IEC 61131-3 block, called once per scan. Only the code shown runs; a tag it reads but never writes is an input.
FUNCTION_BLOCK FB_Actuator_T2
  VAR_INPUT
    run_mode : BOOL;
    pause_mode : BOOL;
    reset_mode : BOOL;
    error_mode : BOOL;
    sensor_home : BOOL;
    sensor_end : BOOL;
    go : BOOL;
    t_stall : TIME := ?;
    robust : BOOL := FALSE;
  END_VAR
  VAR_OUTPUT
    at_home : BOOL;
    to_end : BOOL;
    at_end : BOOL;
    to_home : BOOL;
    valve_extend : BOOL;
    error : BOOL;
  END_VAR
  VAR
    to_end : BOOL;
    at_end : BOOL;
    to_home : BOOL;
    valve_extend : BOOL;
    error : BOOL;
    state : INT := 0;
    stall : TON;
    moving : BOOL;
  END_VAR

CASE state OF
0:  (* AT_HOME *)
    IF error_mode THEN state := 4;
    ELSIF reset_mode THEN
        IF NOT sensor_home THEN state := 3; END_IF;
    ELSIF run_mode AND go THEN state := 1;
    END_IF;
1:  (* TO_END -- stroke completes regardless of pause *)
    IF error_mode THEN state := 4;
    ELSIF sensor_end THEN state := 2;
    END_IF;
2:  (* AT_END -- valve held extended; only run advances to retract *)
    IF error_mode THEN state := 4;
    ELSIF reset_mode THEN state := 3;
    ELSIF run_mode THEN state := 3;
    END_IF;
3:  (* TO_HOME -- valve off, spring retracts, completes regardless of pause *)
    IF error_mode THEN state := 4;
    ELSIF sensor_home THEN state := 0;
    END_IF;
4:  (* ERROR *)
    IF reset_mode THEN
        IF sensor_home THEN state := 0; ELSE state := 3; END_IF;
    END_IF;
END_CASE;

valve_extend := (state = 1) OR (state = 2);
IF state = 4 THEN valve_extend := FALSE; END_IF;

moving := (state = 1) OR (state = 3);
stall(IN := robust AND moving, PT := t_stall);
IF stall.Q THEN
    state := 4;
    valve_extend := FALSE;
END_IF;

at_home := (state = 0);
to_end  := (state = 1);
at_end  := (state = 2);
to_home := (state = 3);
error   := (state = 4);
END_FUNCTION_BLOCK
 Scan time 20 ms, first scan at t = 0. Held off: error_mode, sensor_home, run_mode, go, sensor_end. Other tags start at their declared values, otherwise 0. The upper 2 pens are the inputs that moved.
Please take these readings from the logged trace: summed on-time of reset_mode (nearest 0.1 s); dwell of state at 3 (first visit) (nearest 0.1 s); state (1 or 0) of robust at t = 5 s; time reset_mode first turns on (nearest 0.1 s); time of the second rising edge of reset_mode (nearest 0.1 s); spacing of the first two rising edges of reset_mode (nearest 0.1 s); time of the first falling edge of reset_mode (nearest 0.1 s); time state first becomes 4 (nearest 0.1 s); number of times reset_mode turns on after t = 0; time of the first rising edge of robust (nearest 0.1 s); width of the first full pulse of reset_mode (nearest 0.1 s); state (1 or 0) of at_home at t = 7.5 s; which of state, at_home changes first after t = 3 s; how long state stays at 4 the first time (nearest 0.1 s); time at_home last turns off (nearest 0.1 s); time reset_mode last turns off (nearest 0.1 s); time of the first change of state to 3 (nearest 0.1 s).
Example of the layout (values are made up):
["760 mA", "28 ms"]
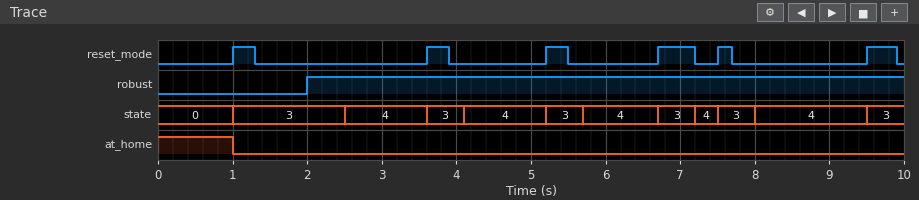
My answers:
["2.0 s", "1.5 s", "1", "1.0 s", "3.6 s", "2.6 s", "1.3 s", "2.5 s", "6", "2.0 s", "0.3 s", "0", "state", "1.1 s", "1.0 s", "9.9 s", "1.0 s"]
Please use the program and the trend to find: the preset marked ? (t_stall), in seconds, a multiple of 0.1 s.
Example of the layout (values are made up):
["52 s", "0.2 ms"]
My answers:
["0.5 s"]
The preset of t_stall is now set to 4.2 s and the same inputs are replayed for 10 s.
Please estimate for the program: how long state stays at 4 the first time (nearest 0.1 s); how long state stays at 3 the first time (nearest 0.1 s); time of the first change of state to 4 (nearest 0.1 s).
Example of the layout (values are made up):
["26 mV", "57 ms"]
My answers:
["0.5 s", "5.2 s", "6.2 s"]
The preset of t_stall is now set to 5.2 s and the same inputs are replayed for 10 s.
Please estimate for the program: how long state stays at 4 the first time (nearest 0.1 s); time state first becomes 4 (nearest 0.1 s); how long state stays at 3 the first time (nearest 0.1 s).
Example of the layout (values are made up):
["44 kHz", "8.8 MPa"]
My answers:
["0.3 s", "7.2 s", "6.2 s"]
